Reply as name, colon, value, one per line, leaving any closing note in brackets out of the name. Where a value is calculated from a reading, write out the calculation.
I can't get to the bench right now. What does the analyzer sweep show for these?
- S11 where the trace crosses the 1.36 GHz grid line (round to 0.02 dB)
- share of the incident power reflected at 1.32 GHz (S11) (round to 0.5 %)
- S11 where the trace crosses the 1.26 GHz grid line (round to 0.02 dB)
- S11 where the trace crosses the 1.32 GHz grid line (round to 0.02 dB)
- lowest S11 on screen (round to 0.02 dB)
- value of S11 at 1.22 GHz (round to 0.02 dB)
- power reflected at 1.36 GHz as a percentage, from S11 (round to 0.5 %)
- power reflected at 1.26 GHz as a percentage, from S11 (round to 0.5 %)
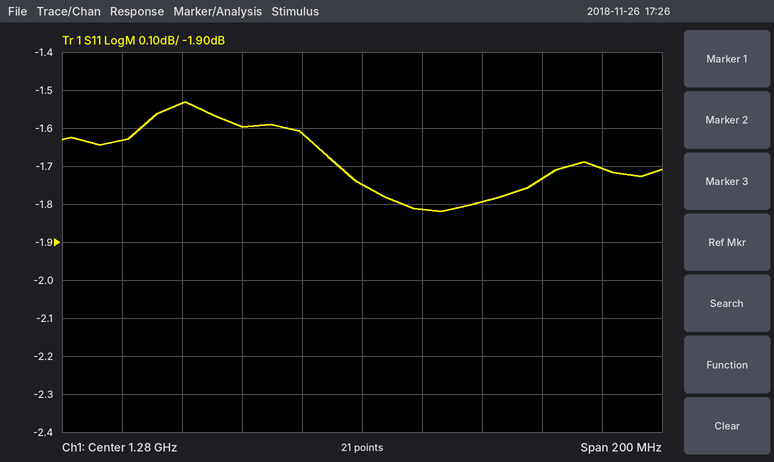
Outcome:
S11 where the trace crosses the 1.36 GHz grid line: -1.70 dB
share of the incident power reflected at 1.32 GHz (S11): 10^(-1.8/10) ≈ 66.1 %, so 66.0 % to the nearest 0.5 %
S11 where the trace crosses the 1.26 GHz grid line: -1.62 dB
S11 where the trace crosses the 1.32 GHz grid line: -1.80 dB
lowest S11 on screen: -1.82 dB
value of S11 at 1.22 GHz: -1.54 dB
power reflected at 1.36 GHz as a percentage, from S11: 10^(-1.7/10) ≈ 67.6 %, so 67.5 % to the nearest 0.5 %
power reflected at 1.26 GHz as a percentage, from S11: 10^(-1.62/10) ≈ 68.9 %, so 69.0 % to the nearest 0.5 %
